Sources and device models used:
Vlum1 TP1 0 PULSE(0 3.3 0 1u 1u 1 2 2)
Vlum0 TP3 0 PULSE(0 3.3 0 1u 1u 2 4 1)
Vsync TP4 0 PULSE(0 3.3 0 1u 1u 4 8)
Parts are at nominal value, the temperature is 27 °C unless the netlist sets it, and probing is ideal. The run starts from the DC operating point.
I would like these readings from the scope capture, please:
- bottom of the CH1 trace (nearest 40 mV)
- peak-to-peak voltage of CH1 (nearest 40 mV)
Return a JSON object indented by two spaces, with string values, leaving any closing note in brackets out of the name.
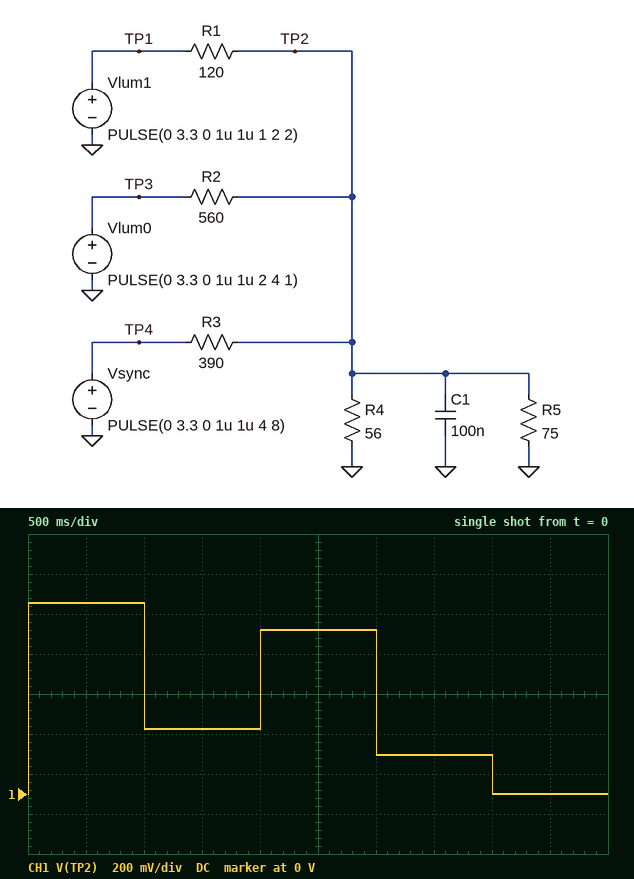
{
  "bottom of the CH1 trace": "0 V",
  "peak-to-peak voltage of CH1": "960 mV"
}
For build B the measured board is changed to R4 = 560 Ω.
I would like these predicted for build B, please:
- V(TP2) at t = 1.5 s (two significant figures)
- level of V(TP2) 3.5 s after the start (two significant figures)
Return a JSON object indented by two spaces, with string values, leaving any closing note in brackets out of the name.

{
  "V(TP2) at t = 1.5 s": "520 mV",
  "level of V(TP2) 3.5 s after the start": "300 mV"
}
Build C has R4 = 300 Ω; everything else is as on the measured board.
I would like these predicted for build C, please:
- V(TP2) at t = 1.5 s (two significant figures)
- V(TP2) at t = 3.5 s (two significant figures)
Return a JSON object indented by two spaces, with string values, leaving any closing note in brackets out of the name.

{
  "V(TP2) at t = 1.5 s": "490 mV",
  "V(TP2) at t = 3.5 s": "290 mV"
}
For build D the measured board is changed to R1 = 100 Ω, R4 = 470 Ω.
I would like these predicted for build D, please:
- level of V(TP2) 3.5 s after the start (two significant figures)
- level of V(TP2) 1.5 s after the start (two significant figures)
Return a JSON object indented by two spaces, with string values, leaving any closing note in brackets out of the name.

{
  "level of V(TP2) 3.5 s after the start": "280 mV",
  "level of V(TP2) 1.5 s after the start": "480 mV"
}
